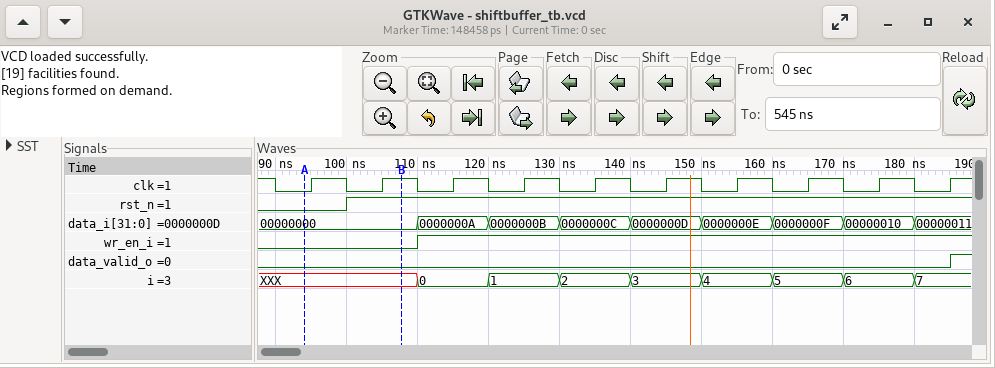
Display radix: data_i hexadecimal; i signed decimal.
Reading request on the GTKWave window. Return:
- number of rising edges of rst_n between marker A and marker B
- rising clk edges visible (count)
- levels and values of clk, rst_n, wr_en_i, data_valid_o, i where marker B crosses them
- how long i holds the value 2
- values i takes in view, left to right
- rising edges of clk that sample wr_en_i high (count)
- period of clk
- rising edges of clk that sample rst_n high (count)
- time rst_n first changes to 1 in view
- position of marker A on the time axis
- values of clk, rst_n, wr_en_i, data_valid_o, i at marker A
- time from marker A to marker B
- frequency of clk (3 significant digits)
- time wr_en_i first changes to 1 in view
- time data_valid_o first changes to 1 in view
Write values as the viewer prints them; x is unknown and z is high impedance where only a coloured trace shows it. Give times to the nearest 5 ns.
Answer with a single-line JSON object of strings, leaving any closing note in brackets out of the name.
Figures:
{"number of rising edges of rst_n between marker A and marker B": "1", "rising clk edges visible": "10", "levels and values of clk, rst_n, wr_en_i, data_valid_o, i where marker B crosses them": "clk=1, rst_n=1, wr_en_i=0, data_valid_o=0, i=XXX", "how long i holds the value 2": "10 ns", "values i takes in view, left to right": "XXX, 0, 1, 2, 3, 4, 5, 6, 7", "rising edges of clk that sample wr_en_i high": "8", "period of clk": "10 ns", "rising edges of clk that sample rst_n high": "9", "time rst_n first changes to 1 in view": "100 ns", "position of marker A on the time axis": "95 ns", "values of clk, rst_n, wr_en_i, data_valid_o, i at marker A": "clk=0, rst_n=0, wr_en_i=0, data_valid_o=0, i=XXX", "time from marker A to marker B": "15 ns", "frequency of clk": "100 MHz", "time wr_en_i first changes to 1 in view": "110 ns", "time data_valid_o first changes to 1 in view": "185 ns"}
